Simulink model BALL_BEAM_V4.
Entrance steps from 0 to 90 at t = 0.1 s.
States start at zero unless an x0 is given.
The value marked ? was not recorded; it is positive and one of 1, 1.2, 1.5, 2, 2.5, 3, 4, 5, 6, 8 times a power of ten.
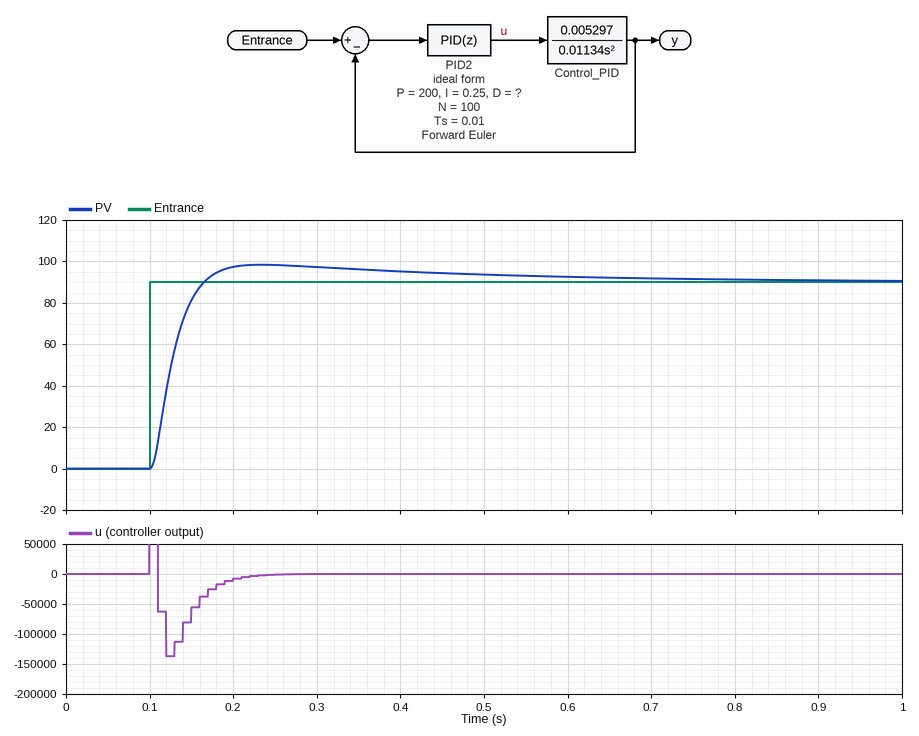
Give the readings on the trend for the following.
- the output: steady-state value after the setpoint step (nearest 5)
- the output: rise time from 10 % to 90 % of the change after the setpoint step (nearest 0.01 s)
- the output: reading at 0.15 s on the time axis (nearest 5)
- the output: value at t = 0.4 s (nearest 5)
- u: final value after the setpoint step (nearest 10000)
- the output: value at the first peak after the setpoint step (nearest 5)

90
0.04 s
80
95
0
100
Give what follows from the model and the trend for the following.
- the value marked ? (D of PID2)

0.3
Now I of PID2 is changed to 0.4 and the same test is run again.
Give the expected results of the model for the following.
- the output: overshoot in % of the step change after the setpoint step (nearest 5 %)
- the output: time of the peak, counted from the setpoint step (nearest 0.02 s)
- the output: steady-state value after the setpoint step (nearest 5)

10 %
0.14 s
90
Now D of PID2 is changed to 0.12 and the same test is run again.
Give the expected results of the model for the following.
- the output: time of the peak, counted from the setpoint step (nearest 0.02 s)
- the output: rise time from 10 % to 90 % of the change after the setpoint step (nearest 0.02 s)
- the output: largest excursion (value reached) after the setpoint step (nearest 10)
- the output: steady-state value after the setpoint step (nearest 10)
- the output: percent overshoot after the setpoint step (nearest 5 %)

0.22 s
0.08 s
120
90
30 %
